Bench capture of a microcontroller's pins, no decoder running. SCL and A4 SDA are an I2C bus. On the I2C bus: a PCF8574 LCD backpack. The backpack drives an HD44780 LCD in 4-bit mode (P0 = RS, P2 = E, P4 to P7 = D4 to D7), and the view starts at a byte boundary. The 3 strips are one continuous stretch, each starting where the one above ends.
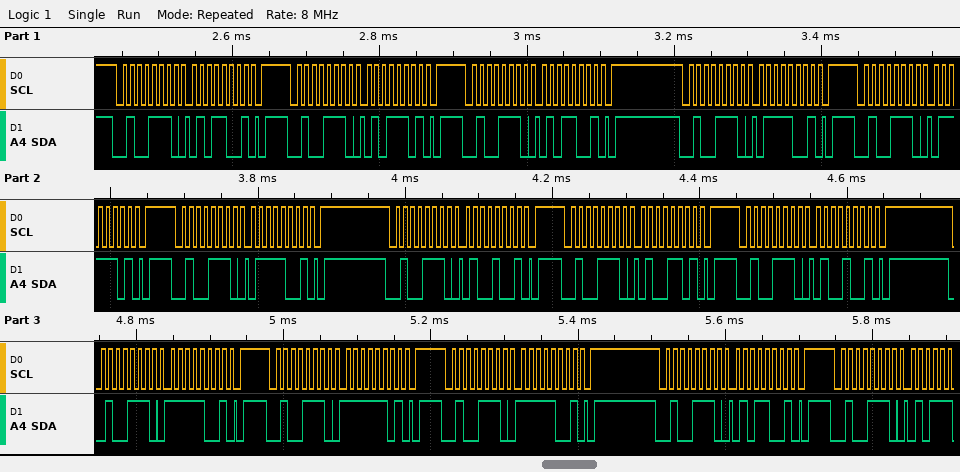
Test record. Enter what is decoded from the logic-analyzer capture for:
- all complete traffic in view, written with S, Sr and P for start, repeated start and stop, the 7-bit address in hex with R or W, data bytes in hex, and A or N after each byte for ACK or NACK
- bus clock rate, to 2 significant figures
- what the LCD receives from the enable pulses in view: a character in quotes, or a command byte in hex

S 27W A 59 A P S 27W A 5D A P S 27W A 59 A P S 27W A 79 A P S 27W A 7D A P S 27W A 79 A P S 27W A 49 A P S 27W A 4D A P S 27W A 49 A P S 27W A F9 A P S 27W A FD A P S 27W A F9 A P S 27W A 59 A P S 27W A
100 kHz
'W' 'O'
